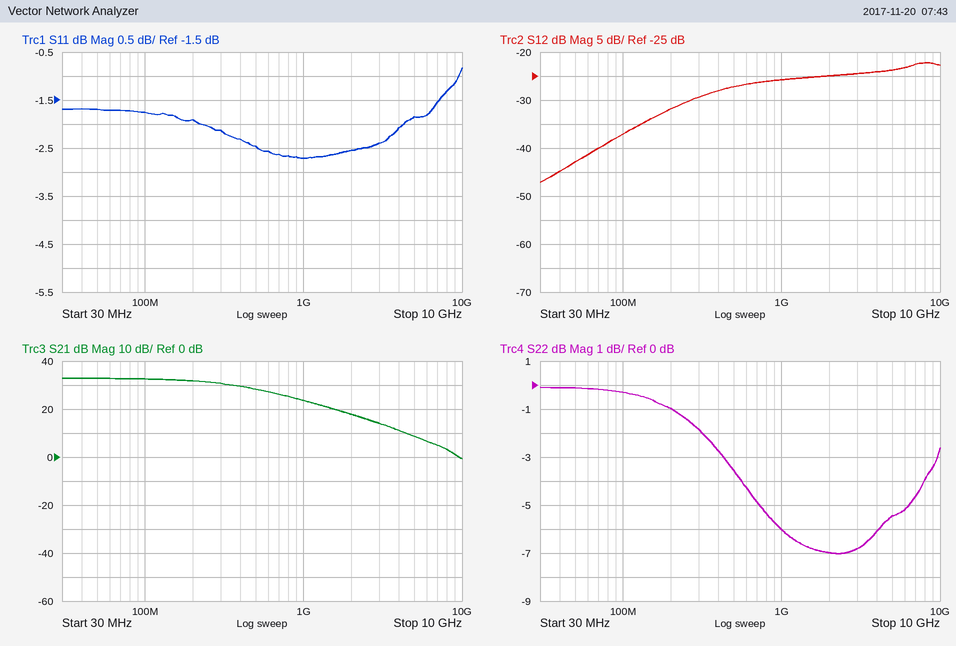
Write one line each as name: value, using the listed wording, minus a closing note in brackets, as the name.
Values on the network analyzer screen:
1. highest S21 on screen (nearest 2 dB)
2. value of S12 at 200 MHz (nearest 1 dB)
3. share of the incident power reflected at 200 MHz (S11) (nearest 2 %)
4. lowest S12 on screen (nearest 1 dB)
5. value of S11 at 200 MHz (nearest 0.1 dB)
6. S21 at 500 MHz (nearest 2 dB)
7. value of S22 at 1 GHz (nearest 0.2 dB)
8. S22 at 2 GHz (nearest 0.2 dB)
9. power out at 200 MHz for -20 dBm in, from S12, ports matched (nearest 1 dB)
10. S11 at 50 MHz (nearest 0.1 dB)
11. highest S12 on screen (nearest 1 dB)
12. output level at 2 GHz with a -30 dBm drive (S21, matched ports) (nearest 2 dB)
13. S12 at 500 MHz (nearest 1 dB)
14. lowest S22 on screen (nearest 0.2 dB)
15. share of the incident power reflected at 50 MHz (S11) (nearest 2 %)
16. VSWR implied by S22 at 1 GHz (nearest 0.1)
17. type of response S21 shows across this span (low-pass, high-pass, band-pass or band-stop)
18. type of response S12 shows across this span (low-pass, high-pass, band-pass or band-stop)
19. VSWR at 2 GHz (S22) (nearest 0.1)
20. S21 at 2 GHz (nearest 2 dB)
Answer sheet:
highest S21 on screen: 32 dB
value of S12 at 200 MHz: -32 dB
share of the incident power reflected at 200 MHz (S11): 64 %
lowest S12 on screen: -47 dB
value of S11 at 200 MHz: -1.9 dB
S21 at 500 MHz: 28 dB
value of S22 at 1 GHz: -6.0 dB
S22 at 2 GHz: -7.0 dB
power out at 200 MHz for -20 dBm in, from S12, ports matched: -52 dBm
S11 at 50 MHz: -1.7 dB
highest S12 on screen: -22 dB
output level at 2 GHz with a -30 dBm drive (S21, matched ports): -12 dBm
S12 at 500 MHz: -27 dB
lowest S22 on screen: -7.0 dB
share of the incident power reflected at 50 MHz (S11): 68 %
VSWR implied by S22 at 1 GHz: 3.0
type of response S21 shows across this span: low-pass
type of response S12 shows across this span: high-pass
VSWR at 2 GHz (S22): 2.6
S21 at 2 GHz: 18 dB
